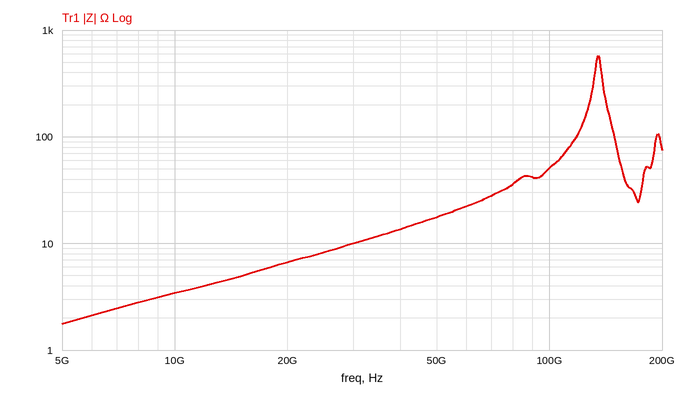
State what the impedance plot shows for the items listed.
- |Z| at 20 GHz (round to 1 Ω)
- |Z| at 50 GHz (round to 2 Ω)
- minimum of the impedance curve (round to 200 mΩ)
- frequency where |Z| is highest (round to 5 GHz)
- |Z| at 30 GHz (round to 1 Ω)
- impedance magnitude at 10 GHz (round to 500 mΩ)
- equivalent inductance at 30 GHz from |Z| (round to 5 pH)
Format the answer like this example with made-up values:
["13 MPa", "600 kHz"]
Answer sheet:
["7 Ω", "18 Ω", "1.8 Ω", "135 GHz", "10 Ω", "3.5 Ω", "55 pH"]
